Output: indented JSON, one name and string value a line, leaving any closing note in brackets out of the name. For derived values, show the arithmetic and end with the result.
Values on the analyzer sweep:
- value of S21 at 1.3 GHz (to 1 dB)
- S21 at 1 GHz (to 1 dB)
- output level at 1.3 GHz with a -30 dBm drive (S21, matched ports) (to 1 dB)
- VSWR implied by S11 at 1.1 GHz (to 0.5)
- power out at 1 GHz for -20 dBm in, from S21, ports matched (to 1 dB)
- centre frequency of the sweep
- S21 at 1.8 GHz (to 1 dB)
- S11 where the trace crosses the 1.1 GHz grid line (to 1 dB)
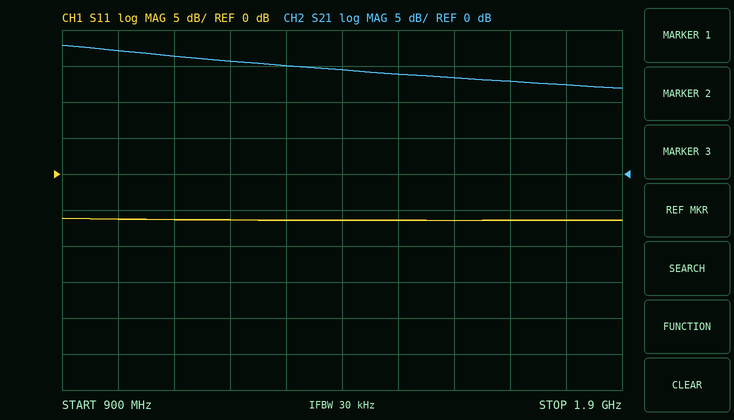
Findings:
{
  "value of S21 at 1.3 GHz": "15 dB",
  "S21 at 1 GHz": "17 dB",
  "output level at 1.3 GHz with a -30 dBm drive (S21, matched ports)": "-30 dBm + (15 dB) = -15 dBm",
  "VSWR implied by S11 at 1.1 GHz": "|Γ| = 10^(-6/20) = 0.5012; VSWR = (1 + 0.5012)/(1 − 0.5012) ≈ 3.0",
  "power out at 1 GHz for -20 dBm in, from S21, ports matched": "-20 dBm + (17 dB) = -3 dBm",
  "centre frequency of the sweep": "1.4 GHz",
  "S21 at 1.8 GHz": "12 dB",
  "S11 where the trace crosses the 1.1 GHz grid line": "-6 dB"
}
